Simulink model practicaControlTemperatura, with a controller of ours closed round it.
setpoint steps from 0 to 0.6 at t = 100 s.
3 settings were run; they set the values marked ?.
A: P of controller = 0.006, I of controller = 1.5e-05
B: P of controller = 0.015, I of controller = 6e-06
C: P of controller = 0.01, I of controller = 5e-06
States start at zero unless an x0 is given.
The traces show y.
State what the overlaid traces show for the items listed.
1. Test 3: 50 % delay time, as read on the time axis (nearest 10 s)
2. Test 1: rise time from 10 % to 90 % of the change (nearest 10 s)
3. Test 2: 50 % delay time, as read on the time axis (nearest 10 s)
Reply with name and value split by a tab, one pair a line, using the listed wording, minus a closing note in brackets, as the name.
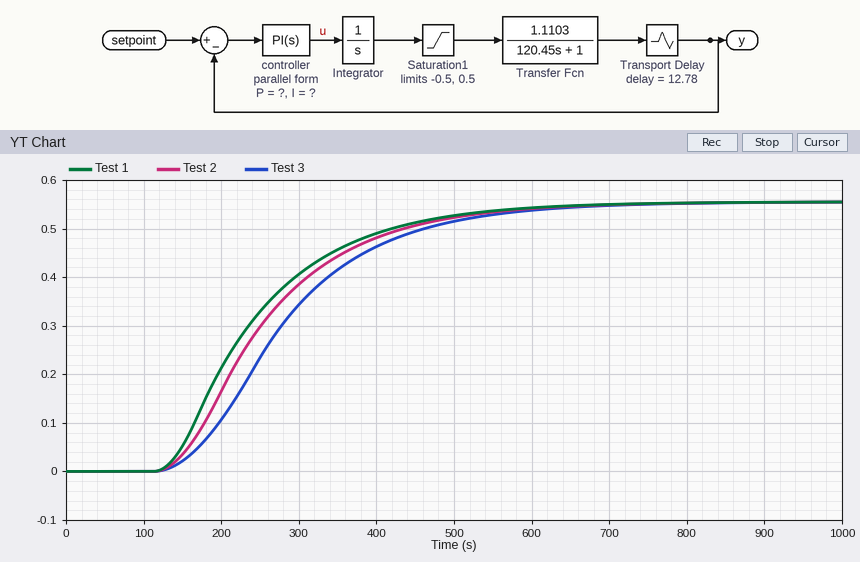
Test 3: 50 % delay time, as read on the time axis	270 s
Test 1: rise time from 10 % to 90 % of the change	270 s
Test 2: 50 % delay time, as read on the time axis	240 s
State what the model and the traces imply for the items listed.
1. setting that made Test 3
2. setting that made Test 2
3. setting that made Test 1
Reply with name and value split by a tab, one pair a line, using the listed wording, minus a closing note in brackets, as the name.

setting that made Test 3	A
setting that made Test 2	C
setting that made Test 1	B
